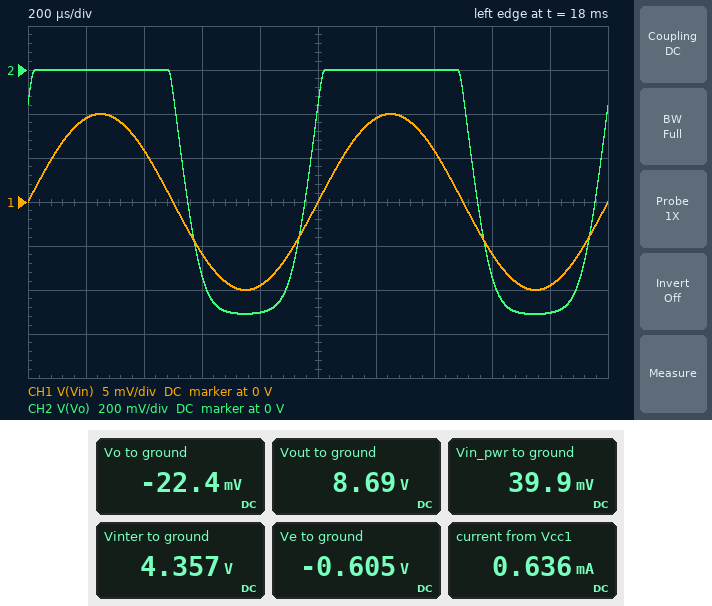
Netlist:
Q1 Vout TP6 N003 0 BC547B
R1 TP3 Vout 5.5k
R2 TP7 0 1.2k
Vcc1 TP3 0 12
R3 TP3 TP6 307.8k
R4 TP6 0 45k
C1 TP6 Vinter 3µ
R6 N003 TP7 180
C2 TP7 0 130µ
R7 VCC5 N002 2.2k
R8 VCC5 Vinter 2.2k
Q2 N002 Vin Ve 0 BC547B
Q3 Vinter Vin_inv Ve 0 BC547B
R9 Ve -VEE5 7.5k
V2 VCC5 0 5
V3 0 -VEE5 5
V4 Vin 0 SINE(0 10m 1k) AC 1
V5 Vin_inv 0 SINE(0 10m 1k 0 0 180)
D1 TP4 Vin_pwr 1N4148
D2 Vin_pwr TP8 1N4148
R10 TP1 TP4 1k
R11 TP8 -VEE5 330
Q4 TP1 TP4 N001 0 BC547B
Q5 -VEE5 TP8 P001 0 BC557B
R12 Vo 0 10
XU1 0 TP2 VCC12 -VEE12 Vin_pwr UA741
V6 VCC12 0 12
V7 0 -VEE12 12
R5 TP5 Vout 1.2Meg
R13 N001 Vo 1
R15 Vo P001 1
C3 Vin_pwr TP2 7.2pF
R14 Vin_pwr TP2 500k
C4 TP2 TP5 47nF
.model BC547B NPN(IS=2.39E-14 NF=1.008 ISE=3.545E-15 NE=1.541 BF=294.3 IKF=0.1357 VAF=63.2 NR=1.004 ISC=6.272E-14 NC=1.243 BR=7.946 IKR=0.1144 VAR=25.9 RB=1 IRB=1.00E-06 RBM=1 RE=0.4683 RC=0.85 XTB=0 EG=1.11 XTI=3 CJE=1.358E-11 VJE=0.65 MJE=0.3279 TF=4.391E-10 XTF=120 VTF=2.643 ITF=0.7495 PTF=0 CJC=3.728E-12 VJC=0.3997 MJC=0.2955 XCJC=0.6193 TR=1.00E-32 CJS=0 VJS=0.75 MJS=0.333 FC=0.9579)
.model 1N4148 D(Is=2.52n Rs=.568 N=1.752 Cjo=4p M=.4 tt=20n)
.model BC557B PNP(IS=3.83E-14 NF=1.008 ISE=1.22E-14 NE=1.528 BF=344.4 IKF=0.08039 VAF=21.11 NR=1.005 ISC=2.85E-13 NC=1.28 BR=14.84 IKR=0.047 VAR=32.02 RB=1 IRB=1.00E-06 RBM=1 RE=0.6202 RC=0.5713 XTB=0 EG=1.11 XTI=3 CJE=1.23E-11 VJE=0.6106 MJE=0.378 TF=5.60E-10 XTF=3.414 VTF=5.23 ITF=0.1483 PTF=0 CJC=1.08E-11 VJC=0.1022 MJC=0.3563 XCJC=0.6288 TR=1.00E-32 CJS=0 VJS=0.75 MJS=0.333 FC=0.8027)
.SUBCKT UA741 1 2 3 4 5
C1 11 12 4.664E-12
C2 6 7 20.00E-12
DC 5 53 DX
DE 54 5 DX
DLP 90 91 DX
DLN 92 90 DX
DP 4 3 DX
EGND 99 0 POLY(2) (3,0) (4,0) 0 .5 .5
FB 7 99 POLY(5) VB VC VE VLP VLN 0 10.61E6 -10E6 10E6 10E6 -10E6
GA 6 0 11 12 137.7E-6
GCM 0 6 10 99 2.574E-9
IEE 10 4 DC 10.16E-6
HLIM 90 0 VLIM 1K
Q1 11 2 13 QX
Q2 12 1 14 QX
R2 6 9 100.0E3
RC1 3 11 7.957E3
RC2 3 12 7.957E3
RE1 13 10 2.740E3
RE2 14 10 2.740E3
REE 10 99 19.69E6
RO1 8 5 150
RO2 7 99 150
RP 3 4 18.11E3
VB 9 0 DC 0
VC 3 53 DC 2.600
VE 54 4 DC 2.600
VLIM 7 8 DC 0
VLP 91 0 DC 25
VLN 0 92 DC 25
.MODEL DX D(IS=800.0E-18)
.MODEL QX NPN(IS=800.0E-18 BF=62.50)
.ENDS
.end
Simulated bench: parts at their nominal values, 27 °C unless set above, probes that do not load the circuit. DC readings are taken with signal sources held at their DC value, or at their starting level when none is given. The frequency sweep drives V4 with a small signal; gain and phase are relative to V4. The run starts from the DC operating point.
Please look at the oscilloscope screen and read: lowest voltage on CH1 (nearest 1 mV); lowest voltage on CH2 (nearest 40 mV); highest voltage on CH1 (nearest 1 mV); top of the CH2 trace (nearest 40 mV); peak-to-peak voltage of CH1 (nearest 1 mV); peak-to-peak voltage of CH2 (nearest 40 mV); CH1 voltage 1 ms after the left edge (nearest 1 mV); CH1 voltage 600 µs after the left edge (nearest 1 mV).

-10 mV
-1.12 V
10 mV
0 V
20 mV
1.12 V
0 V
-6 mV
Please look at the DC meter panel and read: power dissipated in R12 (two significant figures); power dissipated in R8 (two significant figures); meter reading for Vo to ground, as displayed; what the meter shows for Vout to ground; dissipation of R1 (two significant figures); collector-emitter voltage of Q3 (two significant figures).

50 µW
190 µW
-22.4 mV
8.69 V
2.0 mW
5.0 V
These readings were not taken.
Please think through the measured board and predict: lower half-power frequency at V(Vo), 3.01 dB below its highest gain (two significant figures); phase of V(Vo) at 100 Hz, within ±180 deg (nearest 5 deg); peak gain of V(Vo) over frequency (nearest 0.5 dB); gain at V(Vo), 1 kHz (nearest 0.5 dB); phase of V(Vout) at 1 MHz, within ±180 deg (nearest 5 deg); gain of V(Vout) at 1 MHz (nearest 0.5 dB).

8.0 Hz
5 deg
33.5 dB
33.5 dB
145 deg
47.0 dB
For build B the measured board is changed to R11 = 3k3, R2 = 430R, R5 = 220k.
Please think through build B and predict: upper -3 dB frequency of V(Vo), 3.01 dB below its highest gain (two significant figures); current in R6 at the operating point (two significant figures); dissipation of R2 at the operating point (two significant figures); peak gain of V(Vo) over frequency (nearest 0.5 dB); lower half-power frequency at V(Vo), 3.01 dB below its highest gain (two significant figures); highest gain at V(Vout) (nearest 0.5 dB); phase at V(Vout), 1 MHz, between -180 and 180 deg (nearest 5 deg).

40 kHz
1.2 mA
620 µW
26.5 dB
19 Hz
49.0 dB
140 deg
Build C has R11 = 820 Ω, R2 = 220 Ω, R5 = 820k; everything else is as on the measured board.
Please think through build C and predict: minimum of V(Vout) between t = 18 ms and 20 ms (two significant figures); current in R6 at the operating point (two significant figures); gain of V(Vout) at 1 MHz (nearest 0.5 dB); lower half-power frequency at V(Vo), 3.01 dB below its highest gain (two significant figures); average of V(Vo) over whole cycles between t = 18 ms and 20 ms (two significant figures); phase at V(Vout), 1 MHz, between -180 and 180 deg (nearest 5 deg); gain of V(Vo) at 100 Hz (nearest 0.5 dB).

780 mV
1.6 mA
46.5 dB
11 Hz
-840 mV
135 deg
32.0 dB
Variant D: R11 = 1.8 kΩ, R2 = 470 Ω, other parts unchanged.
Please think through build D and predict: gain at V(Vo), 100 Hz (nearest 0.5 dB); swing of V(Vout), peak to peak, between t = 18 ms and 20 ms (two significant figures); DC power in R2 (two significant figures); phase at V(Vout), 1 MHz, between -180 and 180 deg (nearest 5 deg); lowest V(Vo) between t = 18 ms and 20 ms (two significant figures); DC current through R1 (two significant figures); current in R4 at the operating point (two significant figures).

20.0 dB
10 V
610 µW
140 deg
-1.6 V
1.1 mA
31 µA
